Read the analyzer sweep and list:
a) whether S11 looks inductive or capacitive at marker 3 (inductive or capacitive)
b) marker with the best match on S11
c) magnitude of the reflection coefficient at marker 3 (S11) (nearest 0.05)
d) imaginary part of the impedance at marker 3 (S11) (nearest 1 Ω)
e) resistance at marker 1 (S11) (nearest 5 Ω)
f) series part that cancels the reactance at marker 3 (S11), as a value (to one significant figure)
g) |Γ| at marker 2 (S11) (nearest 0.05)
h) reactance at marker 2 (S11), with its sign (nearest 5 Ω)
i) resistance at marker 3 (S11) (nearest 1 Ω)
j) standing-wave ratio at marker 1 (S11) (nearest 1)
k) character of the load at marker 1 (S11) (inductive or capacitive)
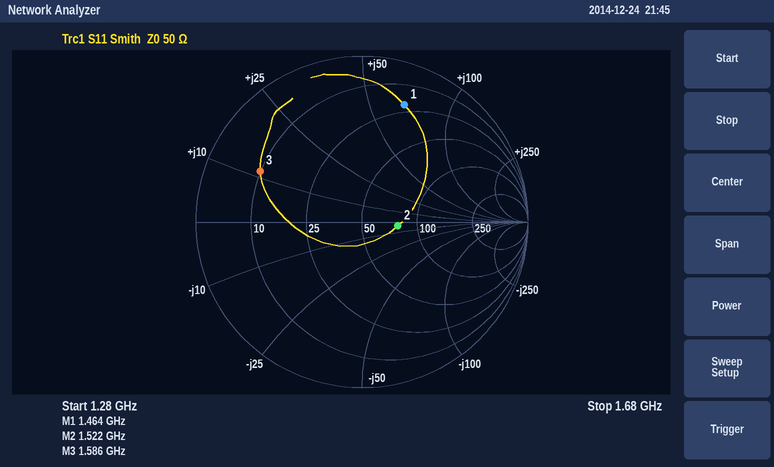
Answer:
inductive
marker 2
0.70
+11 Ω
20 Ω
9 pF
0.20
-5 Ω
10 Ω
7
inductive
